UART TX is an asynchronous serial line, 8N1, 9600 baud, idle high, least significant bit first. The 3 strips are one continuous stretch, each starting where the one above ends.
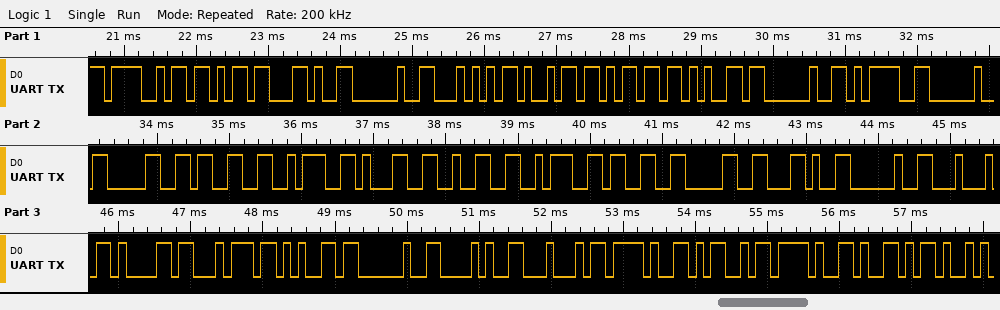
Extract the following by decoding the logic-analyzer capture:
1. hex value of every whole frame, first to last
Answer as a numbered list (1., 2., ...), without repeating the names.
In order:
1. 4F 6B 2C 20 54 69 6D 65 20 3D 20 30 33 3A 31 32 3A 33 30 2C 20 44 61 74 65 20 28 44 2F 4D 2F 59
